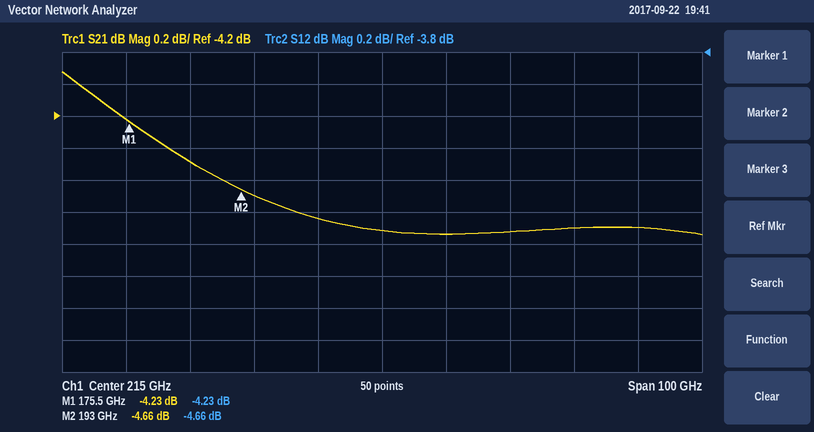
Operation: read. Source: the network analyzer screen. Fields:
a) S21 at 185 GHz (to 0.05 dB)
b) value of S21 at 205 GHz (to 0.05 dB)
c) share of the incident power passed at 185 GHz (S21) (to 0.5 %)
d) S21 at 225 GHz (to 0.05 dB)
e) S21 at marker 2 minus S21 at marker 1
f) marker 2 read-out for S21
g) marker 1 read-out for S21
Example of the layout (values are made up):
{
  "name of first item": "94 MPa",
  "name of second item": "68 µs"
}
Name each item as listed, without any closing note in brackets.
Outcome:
{
  "S21 at 185 GHz": "-4.50 dB",
  "value of S21 at 205 GHz": "-4.85 dB",
  "share of the incident power passed at 185 GHz (S21)": "35.5 %",
  "S21 at 225 GHz": "-4.95 dB",
  "S21 at marker 2 minus S21 at marker 1": "-0.43 dB",
  "marker 2 read-out for S21": "-4.66 dB",
  "marker 1 read-out for S21": "-4.23 dB"
}
